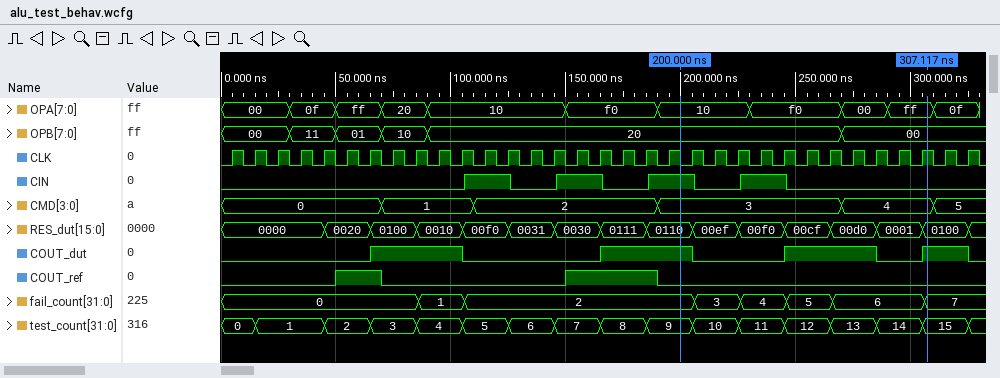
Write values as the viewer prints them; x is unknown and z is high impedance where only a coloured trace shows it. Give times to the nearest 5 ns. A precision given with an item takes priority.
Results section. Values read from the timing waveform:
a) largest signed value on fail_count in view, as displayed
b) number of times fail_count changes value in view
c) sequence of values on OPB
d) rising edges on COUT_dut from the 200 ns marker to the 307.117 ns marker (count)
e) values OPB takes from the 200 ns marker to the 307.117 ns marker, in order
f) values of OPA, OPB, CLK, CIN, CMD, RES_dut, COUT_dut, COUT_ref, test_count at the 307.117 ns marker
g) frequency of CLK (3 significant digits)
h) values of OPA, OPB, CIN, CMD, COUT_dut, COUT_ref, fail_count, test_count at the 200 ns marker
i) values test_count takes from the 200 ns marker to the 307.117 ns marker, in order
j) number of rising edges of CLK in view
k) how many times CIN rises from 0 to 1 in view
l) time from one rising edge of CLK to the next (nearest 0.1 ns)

7
7
00, 11, 01, 10, 20, 00
2
20, 00
OPA=ff, OPB=00, CLK=1, CIN=0, CMD=4, RES_dut=0100, COUT_dut=1, COUT_ref=0, test_count=15
100 MHz
OPA=10, OPB=20, CIN=1, CMD=3, COUT_dut=1, COUT_ref=0, fail_count=2, test_count=9
9, 10, 11, 12, 13, 14, 15
33
4
10 ns
